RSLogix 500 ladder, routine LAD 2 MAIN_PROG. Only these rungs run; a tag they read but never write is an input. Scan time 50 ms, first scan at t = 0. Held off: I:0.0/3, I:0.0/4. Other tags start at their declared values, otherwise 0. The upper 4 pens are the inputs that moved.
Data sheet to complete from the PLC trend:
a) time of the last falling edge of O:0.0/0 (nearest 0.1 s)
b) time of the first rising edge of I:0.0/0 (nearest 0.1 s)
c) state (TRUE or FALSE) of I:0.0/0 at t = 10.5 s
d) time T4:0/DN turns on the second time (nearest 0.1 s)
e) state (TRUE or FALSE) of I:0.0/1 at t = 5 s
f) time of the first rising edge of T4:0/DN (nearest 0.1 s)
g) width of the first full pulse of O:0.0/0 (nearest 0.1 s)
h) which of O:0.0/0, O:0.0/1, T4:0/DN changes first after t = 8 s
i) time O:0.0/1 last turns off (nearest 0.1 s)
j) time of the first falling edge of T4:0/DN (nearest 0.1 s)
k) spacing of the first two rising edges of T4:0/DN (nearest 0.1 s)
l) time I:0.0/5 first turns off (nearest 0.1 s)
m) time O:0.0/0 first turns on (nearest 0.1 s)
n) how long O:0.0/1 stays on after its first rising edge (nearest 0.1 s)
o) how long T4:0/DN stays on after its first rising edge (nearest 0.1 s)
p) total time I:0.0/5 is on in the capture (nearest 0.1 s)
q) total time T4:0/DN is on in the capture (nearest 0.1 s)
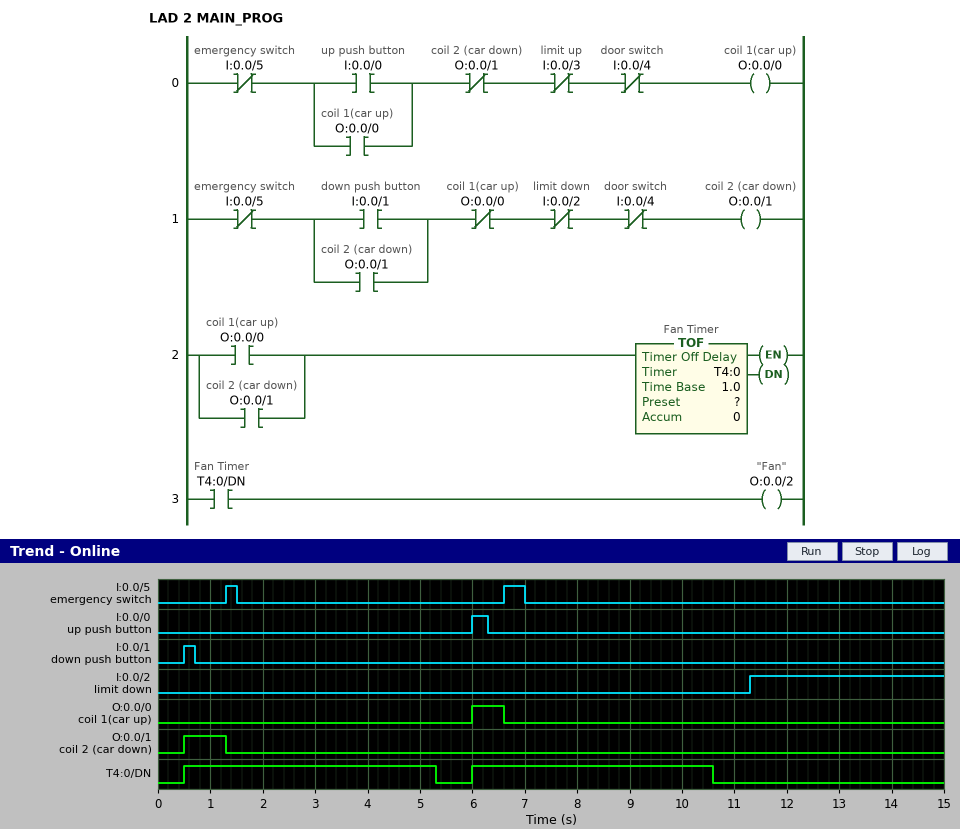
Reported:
6.6 s
6.0 s
FALSE
6.0 s
FALSE
0.5 s
0.6 s
T4:0/DN
1.3 s
5.3 s
5.5 s
1.5 s
6.0 s
0.8 s
4.8 s
0.6 s
9.4 s
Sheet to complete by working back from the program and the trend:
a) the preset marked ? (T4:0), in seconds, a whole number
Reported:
4 s
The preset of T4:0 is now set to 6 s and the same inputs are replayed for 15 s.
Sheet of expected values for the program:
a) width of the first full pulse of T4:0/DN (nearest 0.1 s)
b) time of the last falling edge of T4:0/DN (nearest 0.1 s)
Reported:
12.1 s
12.6 s
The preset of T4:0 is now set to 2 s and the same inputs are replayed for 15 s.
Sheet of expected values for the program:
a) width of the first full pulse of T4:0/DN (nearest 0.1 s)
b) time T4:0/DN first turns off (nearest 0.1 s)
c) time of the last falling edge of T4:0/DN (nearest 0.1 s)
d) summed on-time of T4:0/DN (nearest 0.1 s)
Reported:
2.8 s
3.3 s
8.6 s
5.4 s
